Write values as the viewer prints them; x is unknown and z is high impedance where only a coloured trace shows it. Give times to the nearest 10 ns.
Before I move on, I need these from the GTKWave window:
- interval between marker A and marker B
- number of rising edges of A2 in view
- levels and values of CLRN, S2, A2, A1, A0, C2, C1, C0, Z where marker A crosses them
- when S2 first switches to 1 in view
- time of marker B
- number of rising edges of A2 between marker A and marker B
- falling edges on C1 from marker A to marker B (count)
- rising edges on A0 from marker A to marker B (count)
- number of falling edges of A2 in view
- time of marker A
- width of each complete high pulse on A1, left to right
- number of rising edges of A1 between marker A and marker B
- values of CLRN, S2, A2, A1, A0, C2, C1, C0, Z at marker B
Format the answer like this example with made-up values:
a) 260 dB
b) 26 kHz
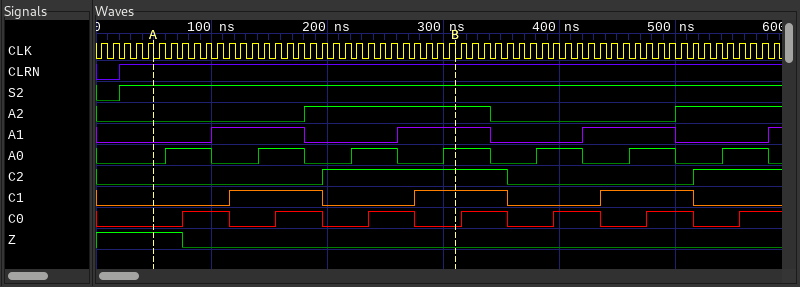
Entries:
a) 260 ns
b) 2
c) CLRN=1, S2=1, A2=0, A1=0, A0=0, C2=0, C1=0, C0=0, Z=1
d) 20 ns
e) 310 ns
f) 1
g) 1
h) 4
i) 1
j) 50 ns
k) 80 ns, 80 ns, 80 ns
l) 2
m) CLRN=1, S2=1, A2=1, A1=1, A0=1, C2=1, C1=1, C0=0, Z=0
